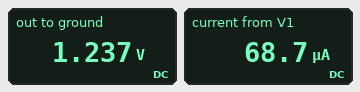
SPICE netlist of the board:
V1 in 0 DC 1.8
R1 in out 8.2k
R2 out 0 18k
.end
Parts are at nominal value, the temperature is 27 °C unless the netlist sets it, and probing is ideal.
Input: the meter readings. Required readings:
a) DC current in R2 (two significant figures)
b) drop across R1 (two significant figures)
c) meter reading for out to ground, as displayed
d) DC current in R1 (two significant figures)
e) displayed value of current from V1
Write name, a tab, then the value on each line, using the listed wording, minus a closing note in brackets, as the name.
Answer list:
DC current in R2	69 µA
drop across R1	560 mV
meter reading for out to ground, as displayed	1.237 V
DC current in R1	69 µA
displayed value of current from V1	68.7 µA
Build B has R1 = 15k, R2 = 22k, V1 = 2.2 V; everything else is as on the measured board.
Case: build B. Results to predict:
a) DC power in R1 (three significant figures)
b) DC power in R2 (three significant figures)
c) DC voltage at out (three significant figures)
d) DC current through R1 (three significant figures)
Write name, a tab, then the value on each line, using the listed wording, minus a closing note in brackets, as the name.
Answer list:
DC power in R1	53.0 µW
DC power in R2	77.8 µW
DC voltage at out	1.31 V
DC current through R1	59.5 µA
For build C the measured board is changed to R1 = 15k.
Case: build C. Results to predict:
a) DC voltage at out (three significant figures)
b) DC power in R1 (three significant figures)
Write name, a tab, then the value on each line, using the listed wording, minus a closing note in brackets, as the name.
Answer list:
DC voltage at out	982 mV
DC power in R1	44.6 µW
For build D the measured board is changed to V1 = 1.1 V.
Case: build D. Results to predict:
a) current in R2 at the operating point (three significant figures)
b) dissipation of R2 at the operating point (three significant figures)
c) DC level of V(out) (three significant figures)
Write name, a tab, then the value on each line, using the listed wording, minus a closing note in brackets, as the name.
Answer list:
current in R2 at the operating point	42.0 µA
dissipation of R2 at the operating point	31.7 µW
DC level of V(out)	756 mV
